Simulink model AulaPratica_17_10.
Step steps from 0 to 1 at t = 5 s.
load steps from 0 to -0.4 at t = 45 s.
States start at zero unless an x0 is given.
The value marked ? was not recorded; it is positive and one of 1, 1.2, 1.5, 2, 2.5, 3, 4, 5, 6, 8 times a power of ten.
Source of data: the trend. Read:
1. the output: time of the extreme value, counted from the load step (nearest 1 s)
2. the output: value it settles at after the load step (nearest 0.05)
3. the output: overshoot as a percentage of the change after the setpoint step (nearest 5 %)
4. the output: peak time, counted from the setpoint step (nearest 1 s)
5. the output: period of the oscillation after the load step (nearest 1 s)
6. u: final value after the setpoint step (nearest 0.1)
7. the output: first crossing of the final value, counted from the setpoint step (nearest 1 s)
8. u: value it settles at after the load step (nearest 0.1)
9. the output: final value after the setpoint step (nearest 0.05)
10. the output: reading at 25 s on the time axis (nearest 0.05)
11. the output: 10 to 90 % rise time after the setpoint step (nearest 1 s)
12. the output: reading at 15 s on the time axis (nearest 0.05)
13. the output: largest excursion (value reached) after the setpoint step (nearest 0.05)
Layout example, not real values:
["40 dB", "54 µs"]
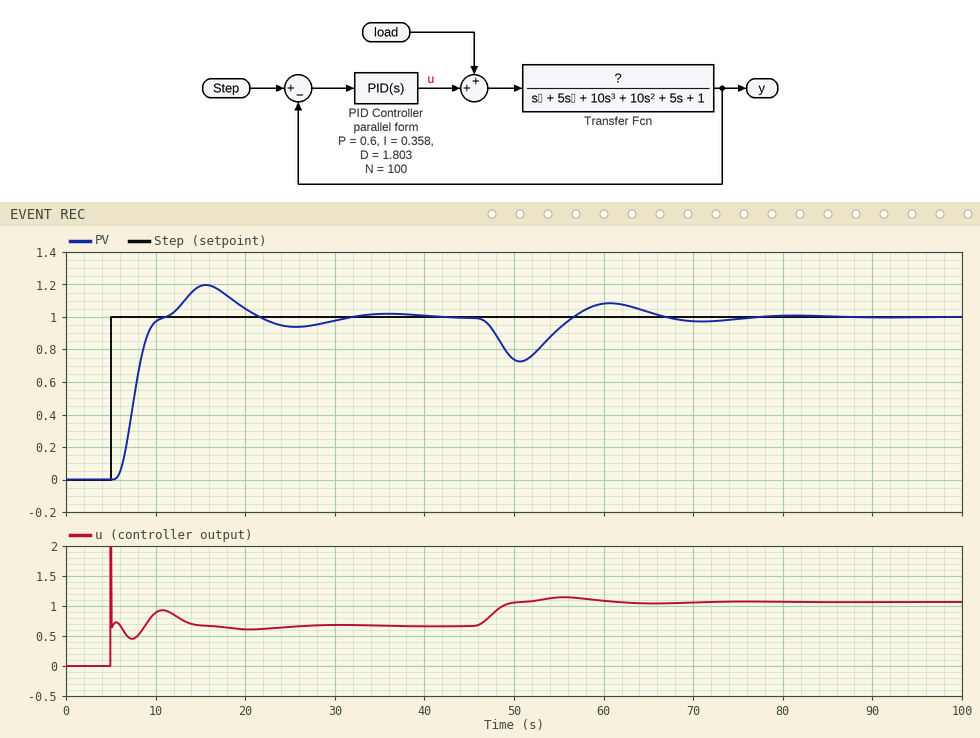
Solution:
["6 s", "1.00", "20 %", "11 s", "20 s", "0.7", "6 s", "1.1", "1.00", "0.95", "3 s", "1.20", "1.20"]
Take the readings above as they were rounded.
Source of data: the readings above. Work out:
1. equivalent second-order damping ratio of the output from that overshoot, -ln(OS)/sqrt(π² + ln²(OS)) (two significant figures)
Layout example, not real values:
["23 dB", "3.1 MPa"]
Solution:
["0.46"]
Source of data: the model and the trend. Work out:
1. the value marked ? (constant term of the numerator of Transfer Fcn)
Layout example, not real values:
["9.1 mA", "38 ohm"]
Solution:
["1.5"]
